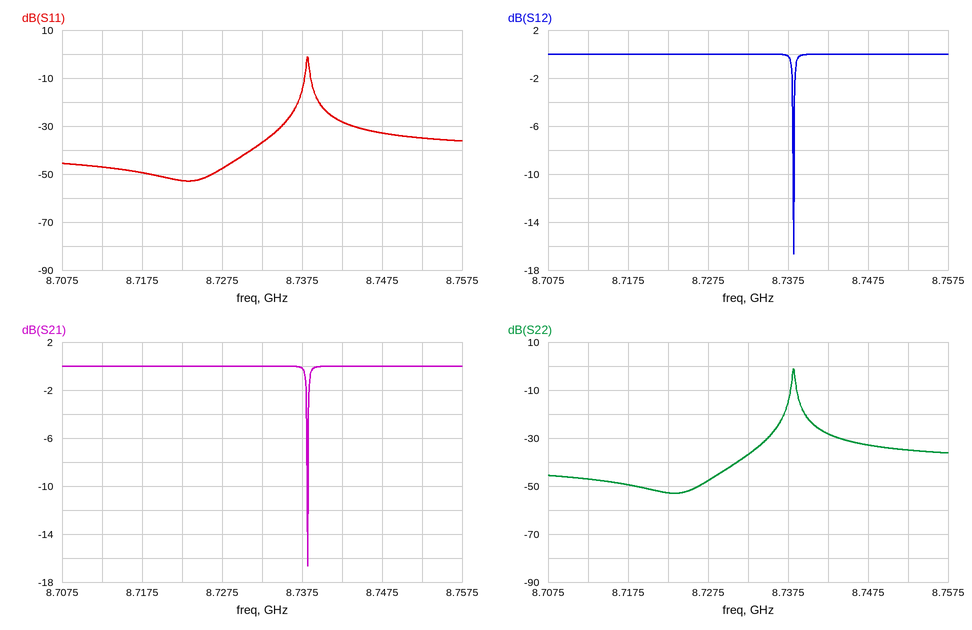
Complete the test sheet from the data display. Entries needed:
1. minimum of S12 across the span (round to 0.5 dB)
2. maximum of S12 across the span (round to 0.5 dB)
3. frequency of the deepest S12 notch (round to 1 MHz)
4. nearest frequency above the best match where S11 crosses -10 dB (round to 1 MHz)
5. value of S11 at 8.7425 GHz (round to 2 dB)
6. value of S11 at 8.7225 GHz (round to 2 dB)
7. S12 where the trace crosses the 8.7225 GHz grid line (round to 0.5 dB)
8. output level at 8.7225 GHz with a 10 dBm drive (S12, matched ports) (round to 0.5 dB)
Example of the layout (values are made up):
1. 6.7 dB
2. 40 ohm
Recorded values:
1. -16.5 dB
2. 0.0 dB
3. 8.738 GHz
4. 8.738 GHz
5. -28 dB
6. -52 dB
7. 0.0 dB
8. 10.0 dBm
